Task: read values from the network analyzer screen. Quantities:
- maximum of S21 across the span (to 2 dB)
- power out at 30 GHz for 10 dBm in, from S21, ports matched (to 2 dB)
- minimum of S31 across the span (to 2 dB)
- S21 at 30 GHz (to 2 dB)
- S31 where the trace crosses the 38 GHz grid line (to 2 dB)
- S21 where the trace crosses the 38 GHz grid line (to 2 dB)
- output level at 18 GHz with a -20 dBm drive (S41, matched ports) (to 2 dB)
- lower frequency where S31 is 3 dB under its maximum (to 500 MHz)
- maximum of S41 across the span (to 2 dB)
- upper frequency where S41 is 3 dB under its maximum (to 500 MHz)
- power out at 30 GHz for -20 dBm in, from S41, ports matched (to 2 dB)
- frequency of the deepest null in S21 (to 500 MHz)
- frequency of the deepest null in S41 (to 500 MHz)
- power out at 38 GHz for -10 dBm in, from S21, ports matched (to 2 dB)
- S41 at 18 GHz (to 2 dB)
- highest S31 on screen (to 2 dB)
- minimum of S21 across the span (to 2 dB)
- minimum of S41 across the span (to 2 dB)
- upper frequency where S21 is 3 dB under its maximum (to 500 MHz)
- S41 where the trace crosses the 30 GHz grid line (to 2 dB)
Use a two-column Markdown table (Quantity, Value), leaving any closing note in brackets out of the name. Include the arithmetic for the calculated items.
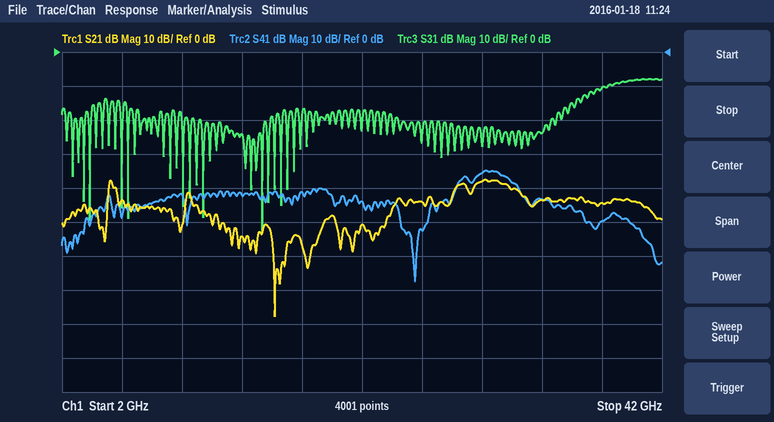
| Quantity | Value |
|---|---|
| maximum of S21 across the span | -38 dB |
| power out at 30 GHz for 10 dBm in, from S21, ports matched | 10 dBm + (-38 dB) = -28 dBm |
| minimum of S31 across the span | -52 dB |
| S21 at 30 GHz | -38 dB |
| S31 where the trace crosses the 38 GHz grid line | -10 dB |
| S21 where the trace crosses the 38 GHz grid line | -44 dB |
| output level at 18 GHz with a -20 dBm drive (S41, matched ports) | -20 dBm + (-42 dB) = -62 dBm |
| lower frequency where S31 is 3 dB under its maximum | 38.0 GHz |
| maximum of S41 across the span | -34 dB |
| upper frequency where S41 is 3 dB under its maximum | 32.0 GHz |
| power out at 30 GHz for -20 dBm in, from S41, ports matched | -20 dBm + (-36 dB) = -56 dBm |
| frequency of the deepest null in S21 | 16.0 GHz |
| frequency of the deepest null in S41 | 25.5 GHz |
| power out at 38 GHz for -10 dBm in, from S21, ports matched | -10 dBm + (-44 dB) = -54 dBm |
| S41 at 18 GHz | -42 dB |
| highest S31 on screen | -8 dB |
| minimum of S21 across the span | -78 dB |
| minimum of S41 across the span | -68 dB |
| upper frequency where S21 is 3 dB under its maximum | 32.5 GHz |
| S41 where the trace crosses the 30 GHz grid line | -36 dB |
